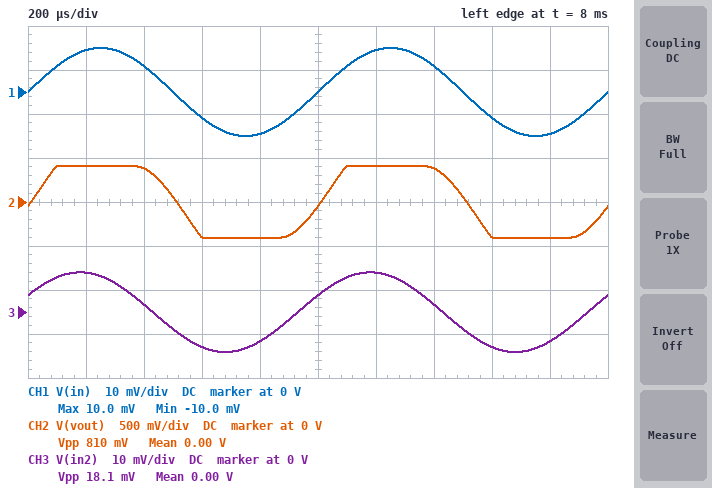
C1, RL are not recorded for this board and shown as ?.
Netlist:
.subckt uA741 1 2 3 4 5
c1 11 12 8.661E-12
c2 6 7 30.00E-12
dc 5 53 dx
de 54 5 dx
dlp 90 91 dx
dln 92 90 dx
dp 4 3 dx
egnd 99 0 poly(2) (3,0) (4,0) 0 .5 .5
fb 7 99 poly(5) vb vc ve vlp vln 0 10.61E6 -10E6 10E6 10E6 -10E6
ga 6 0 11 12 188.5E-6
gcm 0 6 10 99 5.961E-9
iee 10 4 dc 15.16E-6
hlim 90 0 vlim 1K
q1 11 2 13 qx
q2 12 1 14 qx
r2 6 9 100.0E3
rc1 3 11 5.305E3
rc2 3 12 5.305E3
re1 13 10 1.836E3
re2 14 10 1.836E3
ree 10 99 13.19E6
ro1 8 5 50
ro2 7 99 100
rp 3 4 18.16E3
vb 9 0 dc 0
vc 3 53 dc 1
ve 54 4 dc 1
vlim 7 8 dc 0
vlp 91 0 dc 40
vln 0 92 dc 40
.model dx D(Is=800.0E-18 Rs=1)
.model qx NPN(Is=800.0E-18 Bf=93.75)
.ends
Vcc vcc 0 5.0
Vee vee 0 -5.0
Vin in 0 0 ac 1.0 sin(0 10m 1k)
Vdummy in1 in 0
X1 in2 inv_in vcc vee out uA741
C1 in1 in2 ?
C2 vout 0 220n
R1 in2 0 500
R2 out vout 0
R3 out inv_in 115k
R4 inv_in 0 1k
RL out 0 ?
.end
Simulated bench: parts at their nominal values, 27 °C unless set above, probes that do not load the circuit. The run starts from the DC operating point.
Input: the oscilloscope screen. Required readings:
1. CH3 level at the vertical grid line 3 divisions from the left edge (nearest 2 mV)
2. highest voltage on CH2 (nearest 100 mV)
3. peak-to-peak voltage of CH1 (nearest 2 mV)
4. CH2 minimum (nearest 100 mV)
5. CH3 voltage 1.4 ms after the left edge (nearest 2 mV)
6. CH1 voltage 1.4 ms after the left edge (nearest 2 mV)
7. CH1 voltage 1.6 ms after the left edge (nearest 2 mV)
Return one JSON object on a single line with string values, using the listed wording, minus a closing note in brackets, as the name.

{"CH3 level at the vertical grid line 3 divisions from the left edge": "-8 mV", "highest voltage on CH2": "400 mV", "peak-to-peak voltage of CH1": "20 mV", "CH2 minimum": "-400 mV", "CH3 voltage 1.4 ms after the left edge": "2 mV", "CH1 voltage 1.4 ms after the left edge": "6 mV", "CH1 voltage 1.6 ms after the left edge": "-6 mV"}
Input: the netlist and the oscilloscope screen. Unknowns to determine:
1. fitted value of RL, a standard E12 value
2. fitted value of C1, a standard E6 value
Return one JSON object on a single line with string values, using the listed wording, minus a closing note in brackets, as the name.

{"fitted value of RL, a standard E12 value": "10 Ω", "fitted value of C1, a standard E6 value": "680 nF"}
